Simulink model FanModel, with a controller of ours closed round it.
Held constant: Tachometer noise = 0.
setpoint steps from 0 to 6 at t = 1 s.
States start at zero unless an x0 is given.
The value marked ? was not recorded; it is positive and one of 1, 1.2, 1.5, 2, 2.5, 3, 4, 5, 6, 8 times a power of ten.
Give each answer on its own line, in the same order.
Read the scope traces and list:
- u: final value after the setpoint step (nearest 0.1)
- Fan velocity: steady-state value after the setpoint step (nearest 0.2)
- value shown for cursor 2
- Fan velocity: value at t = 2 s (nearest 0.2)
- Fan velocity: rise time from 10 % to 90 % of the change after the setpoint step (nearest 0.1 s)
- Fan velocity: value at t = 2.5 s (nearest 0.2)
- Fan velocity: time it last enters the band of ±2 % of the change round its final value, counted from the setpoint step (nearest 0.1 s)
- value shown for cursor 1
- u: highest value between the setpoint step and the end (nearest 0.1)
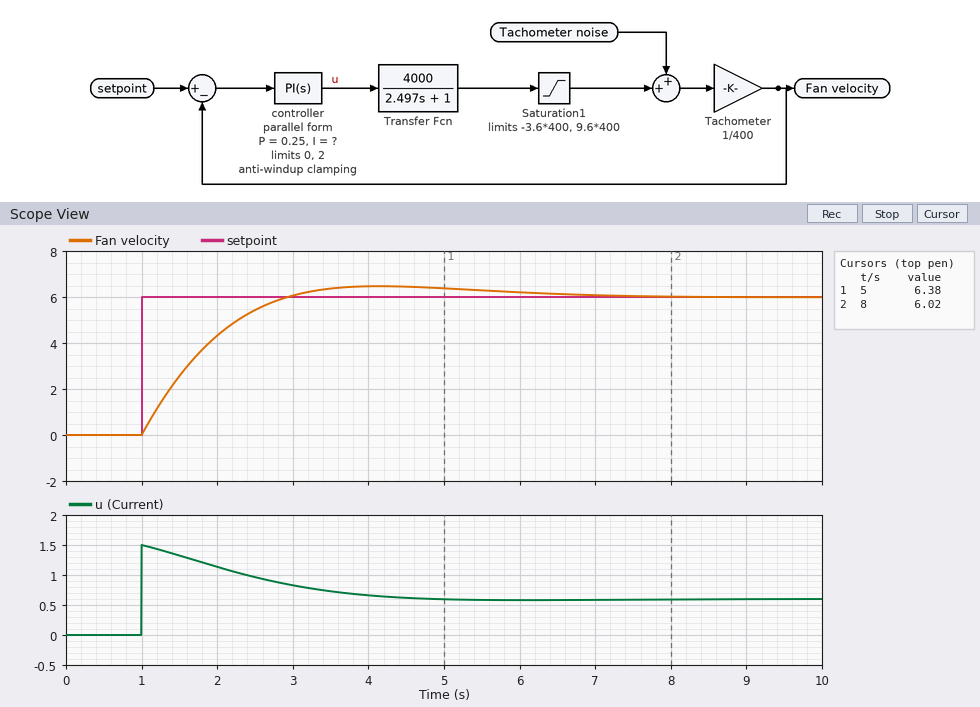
0.6
6.0
6.02
4.4
1.4 s
5.4
5.6 s
6.38
1.5
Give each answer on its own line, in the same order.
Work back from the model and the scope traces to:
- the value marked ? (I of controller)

0.2
